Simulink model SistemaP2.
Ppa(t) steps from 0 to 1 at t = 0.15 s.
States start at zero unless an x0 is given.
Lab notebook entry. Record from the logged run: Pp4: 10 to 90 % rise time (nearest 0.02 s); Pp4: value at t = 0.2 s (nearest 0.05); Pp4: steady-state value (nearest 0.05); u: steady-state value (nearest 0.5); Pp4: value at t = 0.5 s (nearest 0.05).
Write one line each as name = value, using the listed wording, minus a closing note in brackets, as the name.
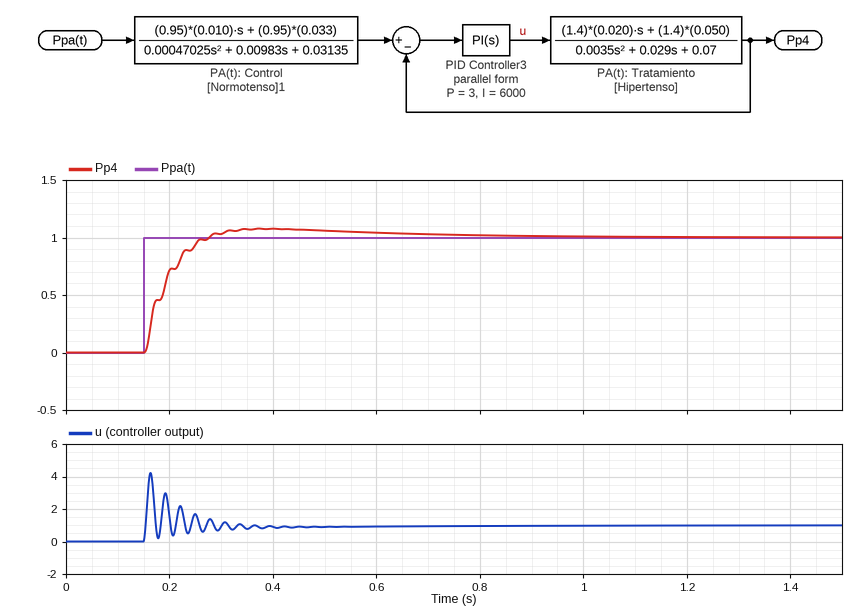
Pp4: 10 to 90 % rise time = 0.08 s
Pp4: value at t = 0.2 s = 0.70
Pp4: steady-state value = 1.00
u: steady-state value = 1.0
Pp4: value at t = 0.5 s = 1.05
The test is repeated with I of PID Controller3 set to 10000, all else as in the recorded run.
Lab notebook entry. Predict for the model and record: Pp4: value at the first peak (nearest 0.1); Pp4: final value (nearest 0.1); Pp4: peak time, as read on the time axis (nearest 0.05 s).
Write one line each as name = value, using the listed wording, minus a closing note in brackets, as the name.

Pp4: value at the first peak = 1.1
Pp4: final value = 1.0
Pp4: peak time, as read on the time axis = 0.40 s
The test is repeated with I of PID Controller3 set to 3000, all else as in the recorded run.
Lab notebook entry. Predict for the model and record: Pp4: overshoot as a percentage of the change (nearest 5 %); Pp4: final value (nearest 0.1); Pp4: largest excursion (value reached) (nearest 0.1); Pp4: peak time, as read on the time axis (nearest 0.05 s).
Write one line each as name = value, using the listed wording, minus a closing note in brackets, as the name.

Pp4: overshoot as a percentage of the change = 10 %
Pp4: final value = 1.0
Pp4: largest excursion (value reached) = 1.1
Pp4: peak time, as read on the time axis = 0.40 s
